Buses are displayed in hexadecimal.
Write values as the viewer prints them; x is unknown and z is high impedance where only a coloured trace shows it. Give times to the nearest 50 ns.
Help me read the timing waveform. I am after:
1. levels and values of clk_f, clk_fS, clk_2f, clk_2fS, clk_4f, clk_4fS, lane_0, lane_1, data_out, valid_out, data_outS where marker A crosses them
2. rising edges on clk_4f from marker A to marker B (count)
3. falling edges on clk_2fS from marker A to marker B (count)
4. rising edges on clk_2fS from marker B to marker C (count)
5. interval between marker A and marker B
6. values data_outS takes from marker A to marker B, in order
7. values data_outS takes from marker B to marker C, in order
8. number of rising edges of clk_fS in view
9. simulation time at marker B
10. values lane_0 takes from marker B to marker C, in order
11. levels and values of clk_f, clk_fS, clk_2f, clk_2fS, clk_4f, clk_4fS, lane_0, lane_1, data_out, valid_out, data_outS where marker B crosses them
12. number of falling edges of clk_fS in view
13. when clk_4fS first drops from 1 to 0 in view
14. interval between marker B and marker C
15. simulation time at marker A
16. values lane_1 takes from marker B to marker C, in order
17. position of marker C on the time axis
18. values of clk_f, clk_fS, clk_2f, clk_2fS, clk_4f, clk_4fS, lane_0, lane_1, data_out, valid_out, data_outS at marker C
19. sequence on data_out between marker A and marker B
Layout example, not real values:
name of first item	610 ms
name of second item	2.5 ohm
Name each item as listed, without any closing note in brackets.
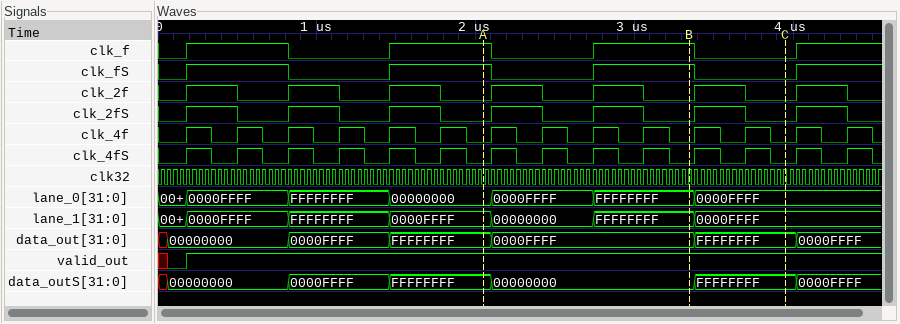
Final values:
levels and values of clk_f, clk_fS, clk_2f, clk_2fS, clk_4f, clk_4fS, lane_0, lane_1, data_out, valid_out, data_outS where marker A crosses them	clk_f=1, clk_fS=1, clk_2f=0, clk_2fS=0, clk_4f=0, clk_4fS=0, lane_0=00000000, lane_1=0000FFFF, data_out=FFFFFFFF, valid_out=1, data_outS=FFFFFFFF
rising edges on clk_4f from marker A to marker B	4
falling edges on clk_2fS from marker A to marker B	2
rising edges on clk_2fS from marker B to marker C	1
interval between marker A and marker B	1300 ns
values data_outS takes from marker A to marker B, in order	FFFFFFFF, 00000000
values data_outS takes from marker B to marker C, in order	00000000, FFFFFFFF
number of rising edges of clk_fS in view	4
simulation time at marker B	3350 ns
values lane_0 takes from marker B to marker C, in order	FFFFFFFF, 0000FFFF
levels and values of clk_f, clk_fS, clk_2f, clk_2fS, clk_4f, clk_4fS, lane_0, lane_1, data_out, valid_out, data_outS where marker B crosses them	clk_f=1, clk_fS=1, clk_2f=0, clk_2fS=0, clk_4f=0, clk_4fS=0, lane_0=FFFFFFFF, lane_1=FFFFFFFF, data_out=0000FFFF, valid_out=1, data_outS=00000000
number of falling edges of clk_fS in view	3
when clk_4fS first drops from 1 to 0 in view	350 ns
interval between marker B and marker C	600 ns
simulation time at marker A	2050 ns
values lane_1 takes from marker B to marker C, in order	FFFFFFFF, 0000FFFF
position of marker C on the time axis	3950 ns
values of clk_f, clk_fS, clk_2f, clk_2fS, clk_4f, clk_4fS, lane_0, lane_1, data_out, valid_out, data_outS at marker C	clk_f=0, clk_fS=0, clk_2f=0, clk_2fS=0, clk_4f=0, clk_4fS=0, lane_0=0000FFFF, lane_1=0000FFFF, data_out=FFFFFFFF, valid_out=1, data_outS=FFFFFFFF
sequence on data_out between marker A and marker B	FFFFFFFF, 0000FFFF
